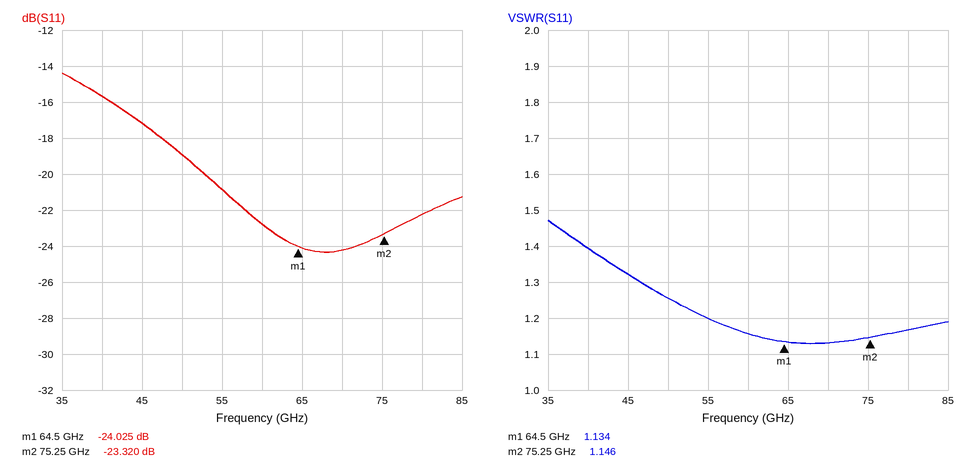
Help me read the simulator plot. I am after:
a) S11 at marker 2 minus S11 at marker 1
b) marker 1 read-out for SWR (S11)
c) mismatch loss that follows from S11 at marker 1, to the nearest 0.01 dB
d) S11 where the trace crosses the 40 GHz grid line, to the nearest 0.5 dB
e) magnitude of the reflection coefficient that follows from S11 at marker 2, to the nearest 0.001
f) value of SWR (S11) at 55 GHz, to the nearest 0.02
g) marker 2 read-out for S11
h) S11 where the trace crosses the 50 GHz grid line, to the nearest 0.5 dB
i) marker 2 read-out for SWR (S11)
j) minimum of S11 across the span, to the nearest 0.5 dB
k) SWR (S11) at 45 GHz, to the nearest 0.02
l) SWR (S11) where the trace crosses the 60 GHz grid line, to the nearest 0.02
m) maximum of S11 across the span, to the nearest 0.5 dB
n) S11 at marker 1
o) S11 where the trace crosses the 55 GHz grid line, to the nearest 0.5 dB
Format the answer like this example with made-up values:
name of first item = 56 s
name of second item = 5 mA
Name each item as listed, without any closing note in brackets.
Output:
S11 at marker 2 minus S11 at marker 1 = 0.705 dB
marker 1 read-out for SWR = 1.134
mismatch loss that follows from S11 at marker 1, to the nearest 0.01 dB = 0.02 dB
S11 where the trace crosses the 40 GHz grid line, to the nearest 0.5 dB = -15.5 dB
magnitude of the reflection coefficient that follows from S11 at marker 2, to the nearest 0.001 = 0.068
value of SWR (S11) at 55 GHz, to the nearest 0.02 = 1.20
marker 2 read-out for S11 = -23.320 dB
S11 where the trace crosses the 50 GHz grid line, to the nearest 0.5 dB = -19.0 dB
marker 2 read-out for SWR = 1.146
minimum of S11 across the span, to the nearest 0.5 dB = -24.5 dB
SWR (S11) at 45 GHz, to the nearest 0.02 = 1.32
SWR (S11) where the trace crosses the 60 GHz grid line, to the nearest 0.02 = 1.16
maximum of S11 across the span, to the nearest 0.5 dB = -14.5 dB
S11 at marker 1 = -24.025 dB
S11 where the trace crosses the 55 GHz grid line, to the nearest 0.5 dB = -21.0 dB
